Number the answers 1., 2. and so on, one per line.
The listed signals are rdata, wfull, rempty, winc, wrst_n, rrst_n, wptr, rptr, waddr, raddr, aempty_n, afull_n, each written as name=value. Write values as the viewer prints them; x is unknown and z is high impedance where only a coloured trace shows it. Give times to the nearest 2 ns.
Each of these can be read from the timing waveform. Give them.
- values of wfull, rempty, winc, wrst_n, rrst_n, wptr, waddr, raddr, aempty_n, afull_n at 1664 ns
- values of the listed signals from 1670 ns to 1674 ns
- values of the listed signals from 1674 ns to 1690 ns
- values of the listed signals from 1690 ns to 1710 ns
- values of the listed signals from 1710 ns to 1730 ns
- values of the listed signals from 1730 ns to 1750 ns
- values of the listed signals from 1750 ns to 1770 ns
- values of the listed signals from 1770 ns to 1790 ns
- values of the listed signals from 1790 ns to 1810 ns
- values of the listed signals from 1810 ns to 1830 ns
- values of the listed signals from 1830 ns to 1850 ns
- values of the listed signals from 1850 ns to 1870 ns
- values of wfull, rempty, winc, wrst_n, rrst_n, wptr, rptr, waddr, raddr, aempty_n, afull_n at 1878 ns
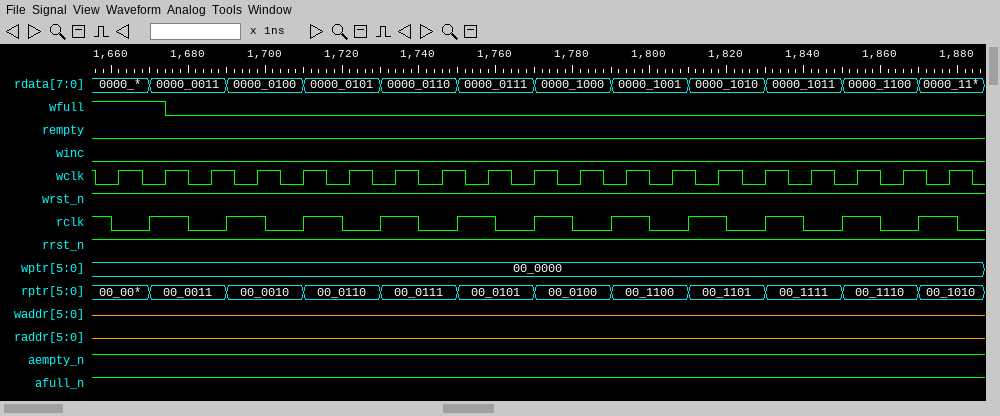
1. wfull=1, rempty=0, winc=0, wrst_n=1, rrst_n=1, wptr=00_0000, waddr=z, raddr=z, aempty_n=1, afull_n=1
2. rdata=0000_0011, wfull=1, rempty=0, winc=0, wrst_n=1, rrst_n=1, wptr=00_0000, rptr=00_0011, waddr=z, raddr=z, aempty_n=1, afull_n=1
3. rdata=0000_0011, wfull=0, rempty=0, winc=0, wrst_n=1, rrst_n=1, wptr=00_0000, rptr=00_0011, waddr=z, raddr=z, aempty_n=1, afull_n=1
4. rdata=0000_0100, wfull=0, rempty=0, winc=0, wrst_n=1, rrst_n=1, wptr=00_0000, rptr=00_0010, waddr=z, raddr=z, aempty_n=1, afull_n=1
5. rdata=0000_0101, wfull=0, rempty=0, winc=0, wrst_n=1, rrst_n=1, wptr=00_0000, rptr=00_0110, waddr=z, raddr=z, aempty_n=1, afull_n=1
6. rdata=0000_0110, wfull=0, rempty=0, winc=0, wrst_n=1, rrst_n=1, wptr=00_0000, rptr=00_0111, waddr=z, raddr=z, aempty_n=1, afull_n=1
7. rdata=0000_0111, wfull=0, rempty=0, winc=0, wrst_n=1, rrst_n=1, wptr=00_0000, rptr=00_0101, waddr=z, raddr=z, aempty_n=1, afull_n=1
8. rdata=0000_1000, wfull=0, rempty=0, winc=0, wrst_n=1, rrst_n=1, wptr=00_0000, rptr=00_0100, waddr=z, raddr=z, aempty_n=1, afull_n=1
9. rdata=0000_1001, wfull=0, rempty=0, winc=0, wrst_n=1, rrst_n=1, wptr=00_0000, rptr=00_1100, waddr=z, raddr=z, aempty_n=1, afull_n=1
10. rdata=0000_1010, wfull=0, rempty=0, winc=0, wrst_n=1, rrst_n=1, wptr=00_0000, rptr=00_1101, waddr=z, raddr=z, aempty_n=1, afull_n=1
11. rdata=0000_1011, wfull=0, rempty=0, winc=0, wrst_n=1, rrst_n=1, wptr=00_0000, rptr=00_1111, waddr=z, raddr=z, aempty_n=1, afull_n=1
12. rdata=0000_1100, wfull=0, rempty=0, winc=0, wrst_n=1, rrst_n=1, wptr=00_0000, rptr=00_1110, waddr=z, raddr=z, aempty_n=1, afull_n=1
13. wfull=0, rempty=0, winc=0, wrst_n=1, rrst_n=1, wptr=00_0000, rptr=00_1010, waddr=z, raddr=z, aempty_n=1, afull_n=1
